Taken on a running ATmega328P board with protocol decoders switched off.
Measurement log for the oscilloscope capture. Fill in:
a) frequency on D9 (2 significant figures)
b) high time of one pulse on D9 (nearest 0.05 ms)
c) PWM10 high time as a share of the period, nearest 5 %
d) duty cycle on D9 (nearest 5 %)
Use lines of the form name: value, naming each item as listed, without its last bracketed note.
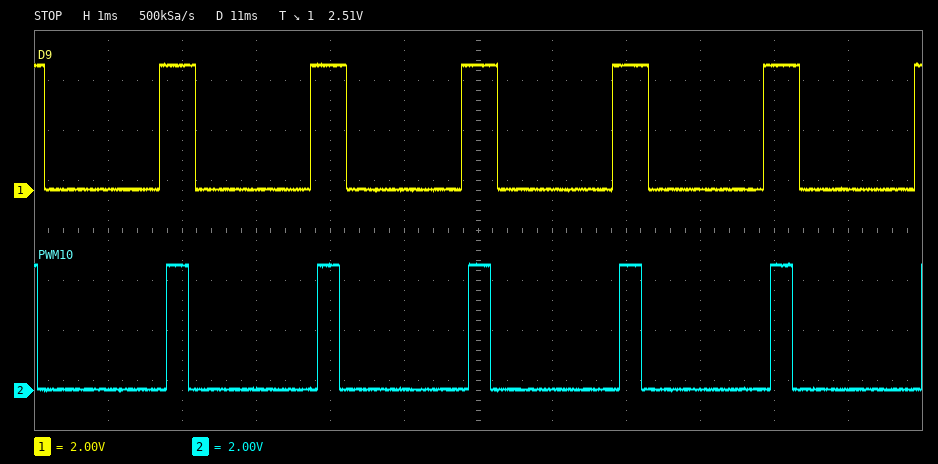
frequency on D9: 490 Hz
high time of one pulse on D9: 0.50 ms
PWM10 high time as a share of the period, nearest 5 %: 15 %
duty cycle on D9: 25 %
